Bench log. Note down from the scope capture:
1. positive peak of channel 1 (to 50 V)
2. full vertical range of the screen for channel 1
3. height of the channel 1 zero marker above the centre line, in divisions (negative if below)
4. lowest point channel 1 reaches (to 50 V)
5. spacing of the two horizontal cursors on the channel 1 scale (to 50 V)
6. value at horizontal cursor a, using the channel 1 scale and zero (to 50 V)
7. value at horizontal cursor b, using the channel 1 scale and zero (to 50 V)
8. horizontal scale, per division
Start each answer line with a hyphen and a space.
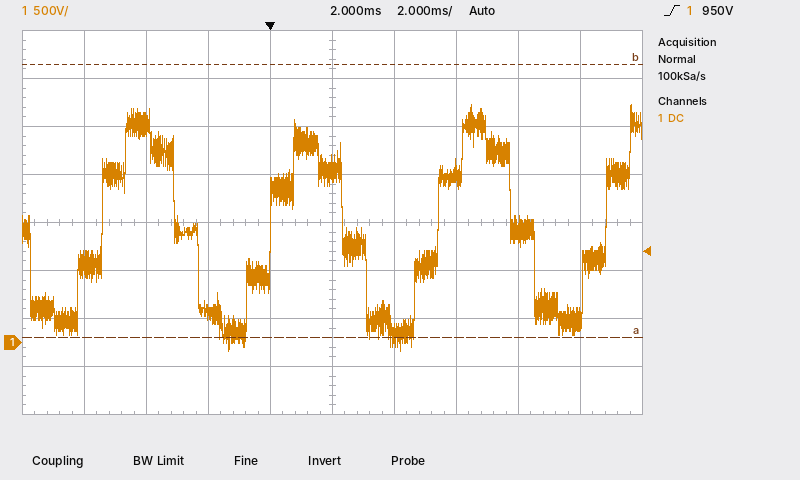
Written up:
- 2.50 kV
- 4 kV
- -2.5 div
- -100 V
- 2.85 kV
- 50 V
- 2.90 kV
- 2 ms
